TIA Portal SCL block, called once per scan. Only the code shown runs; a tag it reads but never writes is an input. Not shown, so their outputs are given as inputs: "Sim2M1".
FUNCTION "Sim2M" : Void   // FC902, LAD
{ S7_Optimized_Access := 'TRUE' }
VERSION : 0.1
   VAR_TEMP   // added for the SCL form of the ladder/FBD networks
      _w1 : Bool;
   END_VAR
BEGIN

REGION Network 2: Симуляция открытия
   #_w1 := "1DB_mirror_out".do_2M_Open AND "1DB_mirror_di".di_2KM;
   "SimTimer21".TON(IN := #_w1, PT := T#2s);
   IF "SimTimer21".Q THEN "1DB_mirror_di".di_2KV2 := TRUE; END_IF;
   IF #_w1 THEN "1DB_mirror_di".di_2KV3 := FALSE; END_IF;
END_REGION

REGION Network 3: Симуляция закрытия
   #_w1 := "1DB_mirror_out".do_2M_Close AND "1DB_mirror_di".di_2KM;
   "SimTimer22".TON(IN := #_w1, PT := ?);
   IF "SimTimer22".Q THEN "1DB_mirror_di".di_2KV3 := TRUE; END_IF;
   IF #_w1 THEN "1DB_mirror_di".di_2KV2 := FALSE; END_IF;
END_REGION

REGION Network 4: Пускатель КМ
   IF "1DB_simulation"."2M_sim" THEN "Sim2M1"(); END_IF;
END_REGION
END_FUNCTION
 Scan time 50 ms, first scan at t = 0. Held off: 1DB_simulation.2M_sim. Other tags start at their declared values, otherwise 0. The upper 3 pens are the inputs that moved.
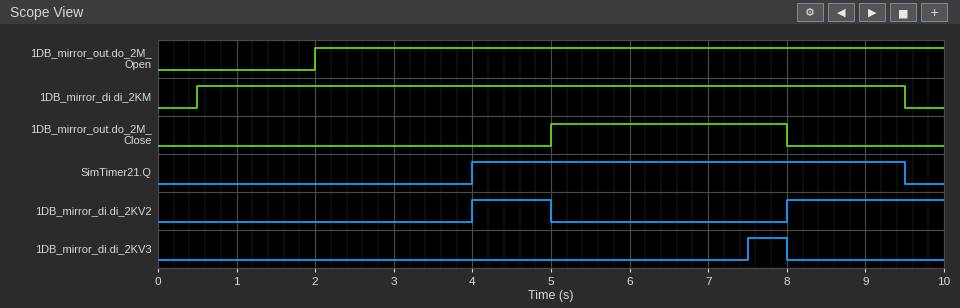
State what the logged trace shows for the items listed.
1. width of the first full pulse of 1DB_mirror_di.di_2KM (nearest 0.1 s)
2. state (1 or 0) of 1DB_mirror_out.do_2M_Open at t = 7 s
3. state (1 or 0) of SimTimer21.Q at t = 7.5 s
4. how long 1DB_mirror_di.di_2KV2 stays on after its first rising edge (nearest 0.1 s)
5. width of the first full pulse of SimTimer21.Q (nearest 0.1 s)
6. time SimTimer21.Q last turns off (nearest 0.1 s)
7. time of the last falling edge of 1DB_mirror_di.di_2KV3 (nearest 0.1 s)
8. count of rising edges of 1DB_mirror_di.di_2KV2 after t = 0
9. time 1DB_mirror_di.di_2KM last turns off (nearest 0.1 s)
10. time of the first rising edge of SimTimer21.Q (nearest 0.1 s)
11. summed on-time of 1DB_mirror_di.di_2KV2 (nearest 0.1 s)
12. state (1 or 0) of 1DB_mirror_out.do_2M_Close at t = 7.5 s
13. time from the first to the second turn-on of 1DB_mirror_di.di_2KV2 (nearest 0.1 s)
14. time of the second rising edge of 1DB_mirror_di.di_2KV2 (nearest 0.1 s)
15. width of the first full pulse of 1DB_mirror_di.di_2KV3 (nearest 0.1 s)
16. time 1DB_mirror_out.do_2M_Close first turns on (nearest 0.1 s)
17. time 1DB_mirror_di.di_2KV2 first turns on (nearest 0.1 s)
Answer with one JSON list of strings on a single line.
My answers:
["9.0 s", "1", "1", "1.0 s", "5.5 s", "9.5 s", "8.0 s", "2", "9.5 s", "4.0 s", "3.0 s", "1", "4.0 s", "8.0 s", "0.5 s", "5.0 s", "4.0 s"]
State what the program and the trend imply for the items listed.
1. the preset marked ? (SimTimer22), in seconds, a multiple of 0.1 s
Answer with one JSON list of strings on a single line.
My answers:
["2.5 s"]
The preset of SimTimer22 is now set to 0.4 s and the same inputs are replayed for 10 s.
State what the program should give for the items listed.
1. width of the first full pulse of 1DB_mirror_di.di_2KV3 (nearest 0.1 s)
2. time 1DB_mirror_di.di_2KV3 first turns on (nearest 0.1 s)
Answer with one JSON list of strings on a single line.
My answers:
["2.6 s", "5.4 s"]
